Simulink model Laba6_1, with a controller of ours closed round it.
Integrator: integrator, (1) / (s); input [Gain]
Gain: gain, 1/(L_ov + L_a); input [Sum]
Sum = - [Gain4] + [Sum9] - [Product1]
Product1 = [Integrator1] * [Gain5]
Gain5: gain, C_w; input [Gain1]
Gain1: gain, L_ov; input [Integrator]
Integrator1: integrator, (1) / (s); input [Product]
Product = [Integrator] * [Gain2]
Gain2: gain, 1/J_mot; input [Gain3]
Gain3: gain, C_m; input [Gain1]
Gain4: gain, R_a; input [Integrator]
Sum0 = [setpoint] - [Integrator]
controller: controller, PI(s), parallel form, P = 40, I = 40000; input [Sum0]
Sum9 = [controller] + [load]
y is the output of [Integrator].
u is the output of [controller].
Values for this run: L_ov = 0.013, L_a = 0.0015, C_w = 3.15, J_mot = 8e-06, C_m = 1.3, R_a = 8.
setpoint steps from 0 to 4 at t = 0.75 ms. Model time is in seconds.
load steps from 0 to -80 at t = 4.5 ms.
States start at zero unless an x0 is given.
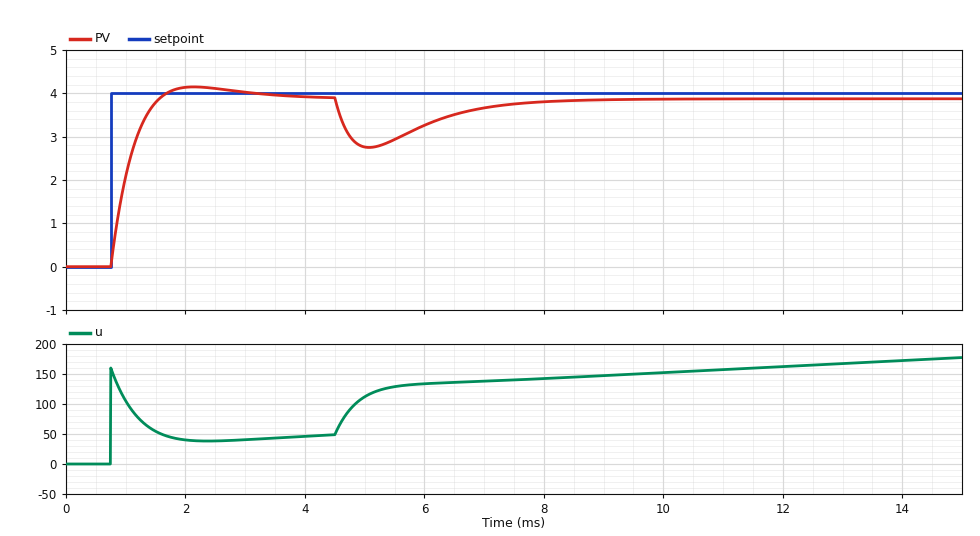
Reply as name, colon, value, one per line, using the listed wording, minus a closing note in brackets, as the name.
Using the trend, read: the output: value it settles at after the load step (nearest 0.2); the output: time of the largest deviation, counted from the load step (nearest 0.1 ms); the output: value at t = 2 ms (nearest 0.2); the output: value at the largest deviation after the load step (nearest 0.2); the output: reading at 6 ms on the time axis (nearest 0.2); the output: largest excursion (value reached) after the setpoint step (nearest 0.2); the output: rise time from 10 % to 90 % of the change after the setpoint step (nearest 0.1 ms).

the output: value it settles at after the load step: 3.8
the output: time of the largest deviation, counted from the load step: 0.6 ms
the output: value at t = 2 ms: 4.2
the output: value at the largest deviation after the load step: 2.8
the output: reading at 6 ms on the time axis: 3.2
the output: largest excursion (value reached) after the setpoint step: 4.2
the output: rise time from 10 % to 90 % of the change after the setpoint step: 0.6 ms
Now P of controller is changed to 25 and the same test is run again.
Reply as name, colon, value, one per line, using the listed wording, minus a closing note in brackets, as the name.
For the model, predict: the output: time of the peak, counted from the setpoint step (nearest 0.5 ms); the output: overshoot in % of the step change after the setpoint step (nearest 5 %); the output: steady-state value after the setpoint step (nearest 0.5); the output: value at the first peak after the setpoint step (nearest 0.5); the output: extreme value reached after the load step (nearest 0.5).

the output: time of the peak, counted from the setpoint step: 1.5 ms
the output: overshoot in % of the step change after the setpoint step: 15 %
the output: steady-state value after the setpoint step: 4.0
the output: value at the first peak after the setpoint step: 4.5
the output: extreme value reached after the load step: 2.5
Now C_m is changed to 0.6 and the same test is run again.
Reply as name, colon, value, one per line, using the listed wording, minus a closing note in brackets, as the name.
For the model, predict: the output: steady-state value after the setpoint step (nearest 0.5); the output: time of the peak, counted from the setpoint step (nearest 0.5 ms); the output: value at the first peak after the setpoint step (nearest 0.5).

the output: steady-state value after the setpoint step: 4.0
the output: time of the peak, counted from the setpoint step: 1.5 ms
the output: value at the first peak after the setpoint step: 4.0
